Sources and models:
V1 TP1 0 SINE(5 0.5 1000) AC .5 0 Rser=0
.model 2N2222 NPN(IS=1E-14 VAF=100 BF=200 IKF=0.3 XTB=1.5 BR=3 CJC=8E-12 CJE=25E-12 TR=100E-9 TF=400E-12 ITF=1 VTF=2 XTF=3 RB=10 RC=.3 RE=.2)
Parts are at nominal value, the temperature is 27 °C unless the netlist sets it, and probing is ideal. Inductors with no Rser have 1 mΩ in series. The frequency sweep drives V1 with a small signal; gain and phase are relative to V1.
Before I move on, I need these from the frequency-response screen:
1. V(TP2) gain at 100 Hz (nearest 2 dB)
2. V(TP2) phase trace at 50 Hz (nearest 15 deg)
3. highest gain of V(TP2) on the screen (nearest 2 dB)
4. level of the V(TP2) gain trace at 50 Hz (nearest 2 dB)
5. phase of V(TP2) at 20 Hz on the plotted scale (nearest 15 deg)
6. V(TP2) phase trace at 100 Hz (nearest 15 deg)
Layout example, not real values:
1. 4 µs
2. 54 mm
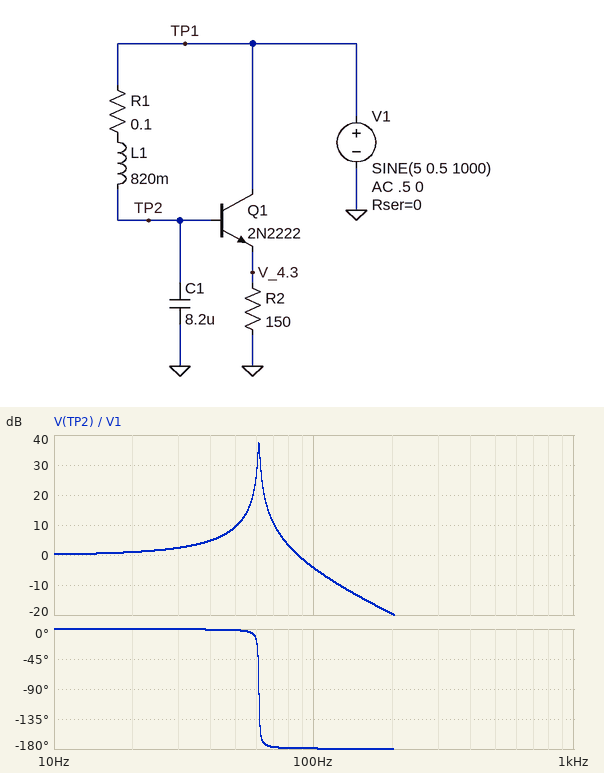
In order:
1. -4 dB
2. 0 deg
3. 38 dB
4. 10 dB
5. 0 deg
6. -180 deg
